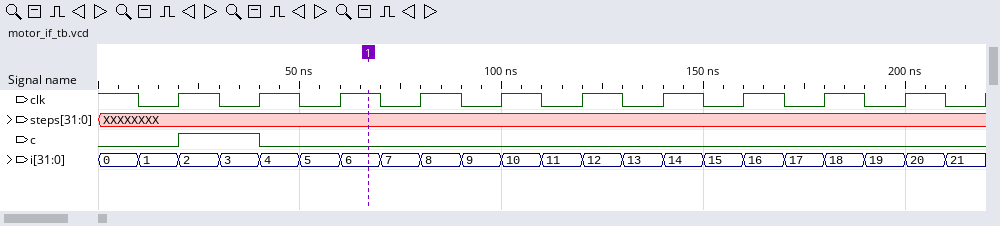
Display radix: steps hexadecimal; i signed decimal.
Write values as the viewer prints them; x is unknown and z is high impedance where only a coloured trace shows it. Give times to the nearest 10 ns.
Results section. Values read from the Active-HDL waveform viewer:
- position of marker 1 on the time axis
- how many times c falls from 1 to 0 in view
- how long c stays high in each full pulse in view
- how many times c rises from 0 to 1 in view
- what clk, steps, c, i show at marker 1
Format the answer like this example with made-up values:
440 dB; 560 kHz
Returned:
70 ns; 1; 20 ns; 1; clk=1, steps=XXXXXXXX, c=0, i=6
